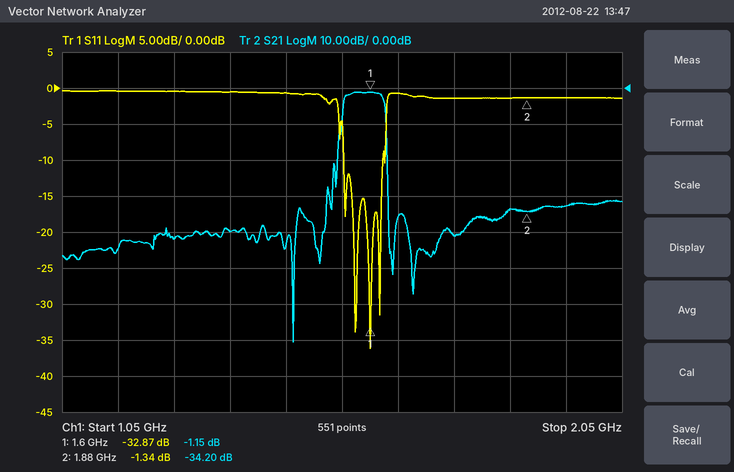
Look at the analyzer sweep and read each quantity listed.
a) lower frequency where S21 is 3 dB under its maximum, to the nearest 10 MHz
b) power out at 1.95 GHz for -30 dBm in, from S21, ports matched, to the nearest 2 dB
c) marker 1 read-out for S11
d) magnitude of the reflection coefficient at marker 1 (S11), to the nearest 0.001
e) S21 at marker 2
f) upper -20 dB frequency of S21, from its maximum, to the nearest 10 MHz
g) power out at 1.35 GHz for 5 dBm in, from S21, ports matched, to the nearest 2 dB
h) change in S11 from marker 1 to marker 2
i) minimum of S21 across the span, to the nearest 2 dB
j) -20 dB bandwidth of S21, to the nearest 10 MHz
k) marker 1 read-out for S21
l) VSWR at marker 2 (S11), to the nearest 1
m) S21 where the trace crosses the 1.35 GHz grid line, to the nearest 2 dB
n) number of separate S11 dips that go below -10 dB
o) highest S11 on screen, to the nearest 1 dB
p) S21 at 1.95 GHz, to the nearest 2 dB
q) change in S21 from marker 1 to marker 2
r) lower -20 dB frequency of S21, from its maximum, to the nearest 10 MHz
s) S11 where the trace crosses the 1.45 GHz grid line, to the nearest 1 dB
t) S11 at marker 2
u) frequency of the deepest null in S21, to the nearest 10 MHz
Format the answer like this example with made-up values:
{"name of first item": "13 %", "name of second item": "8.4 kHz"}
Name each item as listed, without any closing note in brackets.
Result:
{"lower frequency where S21 is 3 dB under its maximum, to the nearest 10 MHz": "1.55 GHz", "power out at 1.95 GHz for -30 dBm in, from S21, ports matched, to the nearest 2 dB": "-62 dBm", "marker 1 read-out for S11": "-32.87 dB", "magnitude of the reflection coefficient at marker 1 (S11), to the nearest 0.001": "0.023", "S21 at marker 2": "-34.20 dB", "upper -20 dB frequency of S21, from its maximum, to the nearest 10 MHz": "1.63 GHz", "power out at 1.35 GHz for 5 dBm in, from S21, ports matched, to the nearest 2 dB": "-34 dBm", "change in S11 from marker 1 to marker 2": "31.53 dB", "minimum of S21 across the span, to the nearest 2 dB": "-70 dB", "-20 dB bandwidth of S21, to the nearest 10 MHz": "90 MHz", "marker 1 read-out for S21": "-1.15 dB", "VSWR at marker 2 (S11), to the nearest 1": "13", "S21 where the trace crosses the 1.35 GHz grid line, to the nearest 2 dB": "-40 dB", "number of separate S11 dips that go below -10 dB": "4", "highest S11 on screen, to the nearest 1 dB": "0 dB", "S21 at 1.95 GHz, to the nearest 2 dB": "-32 dB", "change in S21 from marker 1 to marker 2": "-33.05 dB", "lower -20 dB frequency of S21, from its maximum, to the nearest 10 MHz": "1.54 GHz", "S11 where the trace crosses the 1.45 GHz grid line, to the nearest 1 dB": "-1 dB", "S11 at marker 2": "-1.34 dB", "frequency of the deepest null in S21, to the nearest 10 MHz": "1.46 GHz"}
